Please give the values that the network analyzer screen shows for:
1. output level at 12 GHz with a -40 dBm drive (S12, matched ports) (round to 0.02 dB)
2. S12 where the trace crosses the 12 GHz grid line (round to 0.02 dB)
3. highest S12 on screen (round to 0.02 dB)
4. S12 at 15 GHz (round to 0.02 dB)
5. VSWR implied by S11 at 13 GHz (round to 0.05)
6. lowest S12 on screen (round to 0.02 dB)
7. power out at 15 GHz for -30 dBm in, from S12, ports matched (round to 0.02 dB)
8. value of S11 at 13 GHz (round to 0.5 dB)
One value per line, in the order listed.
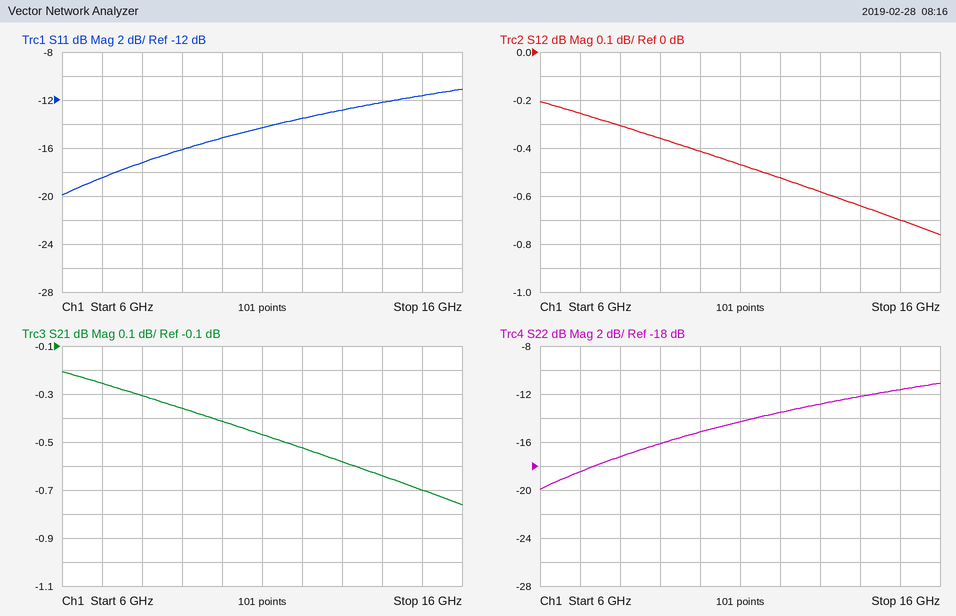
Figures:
-40.52 dBm
-0.52 dB
-0.20 dB
-0.70 dB
1.60
-0.76 dB
-30.70 dBm
-13.0 dB
